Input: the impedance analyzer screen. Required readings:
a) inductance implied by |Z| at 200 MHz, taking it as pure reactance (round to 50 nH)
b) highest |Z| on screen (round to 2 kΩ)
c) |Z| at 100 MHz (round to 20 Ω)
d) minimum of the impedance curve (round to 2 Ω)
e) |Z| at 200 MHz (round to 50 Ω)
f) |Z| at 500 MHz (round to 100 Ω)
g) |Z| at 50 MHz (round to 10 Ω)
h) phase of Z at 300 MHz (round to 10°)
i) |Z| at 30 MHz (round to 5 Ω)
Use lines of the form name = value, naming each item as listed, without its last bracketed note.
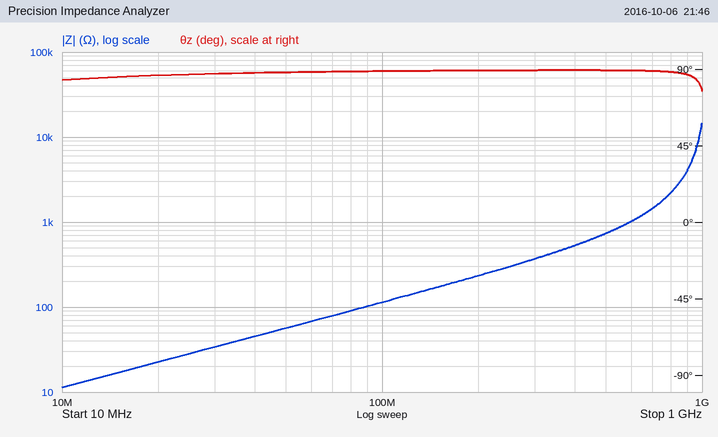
inductance implied by |Z| at 200 MHz, taking it as pure reactance = 200 nH
highest |Z| on screen = 14 kΩ
|Z| at 100 MHz = 120 Ω
minimum of the impedance curve = 12 Ω
|Z| at 200 MHz = 250 Ω
|Z| at 500 MHz = 700 Ω
|Z| at 50 MHz = 60 Ω
phase of Z at 300 MHz = 90°
|Z| at 30 MHz = 35 Ω
